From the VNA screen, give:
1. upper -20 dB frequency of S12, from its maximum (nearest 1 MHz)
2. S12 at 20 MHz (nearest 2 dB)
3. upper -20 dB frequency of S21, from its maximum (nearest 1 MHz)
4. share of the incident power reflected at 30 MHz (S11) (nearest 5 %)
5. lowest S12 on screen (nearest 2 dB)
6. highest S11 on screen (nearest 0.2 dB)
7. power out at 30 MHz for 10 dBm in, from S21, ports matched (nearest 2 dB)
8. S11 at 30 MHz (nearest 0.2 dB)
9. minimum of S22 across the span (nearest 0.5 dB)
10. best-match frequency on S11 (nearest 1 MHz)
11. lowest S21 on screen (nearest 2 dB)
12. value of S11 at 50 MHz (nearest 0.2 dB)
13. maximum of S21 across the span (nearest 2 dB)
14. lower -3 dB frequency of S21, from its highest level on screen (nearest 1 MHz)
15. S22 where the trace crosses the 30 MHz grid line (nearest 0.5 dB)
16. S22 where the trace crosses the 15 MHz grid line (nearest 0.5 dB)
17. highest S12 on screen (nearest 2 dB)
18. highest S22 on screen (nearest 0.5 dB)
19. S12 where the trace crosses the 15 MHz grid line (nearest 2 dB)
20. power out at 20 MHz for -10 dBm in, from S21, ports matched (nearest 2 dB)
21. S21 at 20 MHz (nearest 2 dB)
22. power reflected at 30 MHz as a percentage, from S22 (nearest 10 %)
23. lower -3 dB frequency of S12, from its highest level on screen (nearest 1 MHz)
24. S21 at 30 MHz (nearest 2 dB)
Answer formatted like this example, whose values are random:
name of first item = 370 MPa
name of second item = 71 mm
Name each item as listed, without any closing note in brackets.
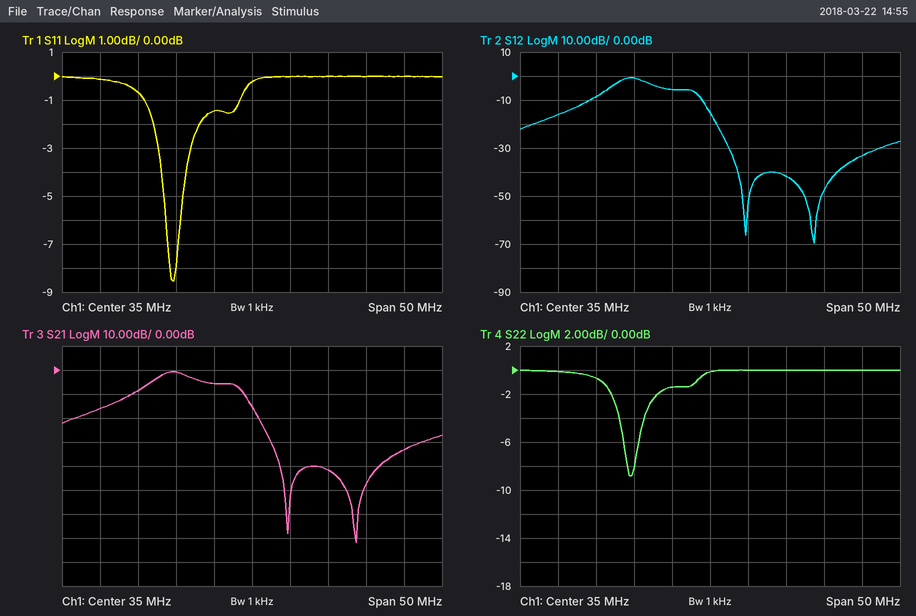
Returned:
upper -20 dB frequency of S12, from its maximum = 36 MHz
S12 at 20 MHz = -8 dB
upper -20 dB frequency of S21, from its maximum = 36 MHz
share of the incident power reflected at 30 MHz (S11) = 70 %
lowest S12 on screen = -70 dB
highest S11 on screen = 0.0 dB
power out at 30 MHz for 10 dBm in, from S21, ports matched = 4 dBm
S11 at 30 MHz = -1.4 dB
minimum of S22 across the span = -9.0 dB
best-match frequency on S11 = 25 MHz
lowest S21 on screen = -72 dB
value of S11 at 50 MHz = 0.0 dB
maximum of S21 across the span = 0 dB
lower -3 dB frequency of S21, from its highest level on screen = 22 MHz
S22 where the trace crosses the 30 MHz grid line = -1.5 dB
S22 where the trace crosses the 15 MHz grid line = 0.0 dB
highest S12 on screen = 0 dB
highest S22 on screen = 0.0 dB
S12 where the trace crosses the 15 MHz grid line = -16 dB
power out at 20 MHz for -10 dBm in, from S21, ports matched = -18 dBm
S21 at 20 MHz = -8 dB
power reflected at 30 MHz as a percentage, from S22 = 70 %
lower -3 dB frequency of S12, from its highest level on screen = 22 MHz
S21 at 30 MHz = -6 dB
